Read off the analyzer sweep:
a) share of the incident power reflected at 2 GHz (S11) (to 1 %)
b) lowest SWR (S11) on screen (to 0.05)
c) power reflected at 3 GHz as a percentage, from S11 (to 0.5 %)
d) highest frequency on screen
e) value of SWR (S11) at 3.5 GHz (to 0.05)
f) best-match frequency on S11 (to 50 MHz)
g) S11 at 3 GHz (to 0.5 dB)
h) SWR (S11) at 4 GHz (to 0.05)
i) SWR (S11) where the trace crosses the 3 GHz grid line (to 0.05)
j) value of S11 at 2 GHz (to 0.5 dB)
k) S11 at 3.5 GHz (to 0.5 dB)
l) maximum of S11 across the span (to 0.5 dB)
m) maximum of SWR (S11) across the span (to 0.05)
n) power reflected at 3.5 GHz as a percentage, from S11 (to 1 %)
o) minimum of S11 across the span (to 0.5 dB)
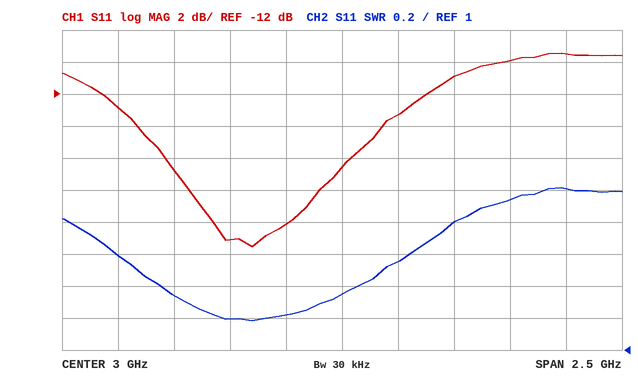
5 %
1.20
2.0 %
4.25 GHz
1.80
2.60 GHz
-16.5 dB
2.00
1.35
-13.0 dB
-11.0 dB
-9.5 dB
2.00
8 %
-21.5 dB
